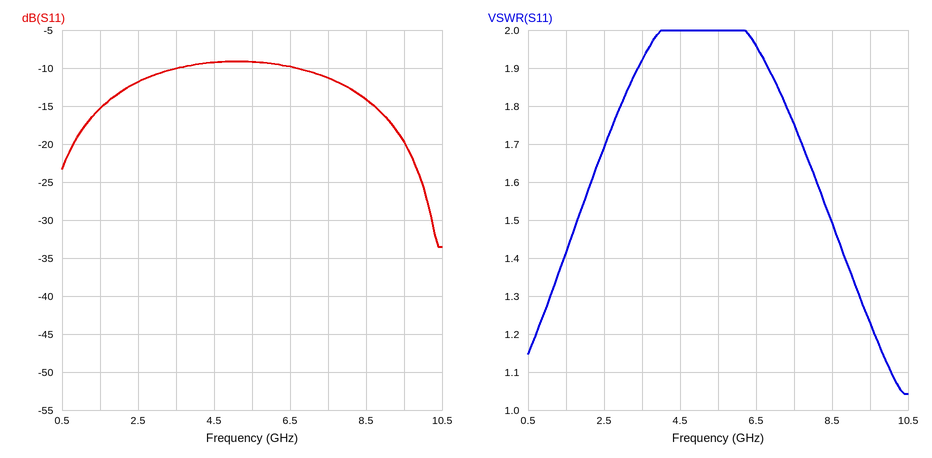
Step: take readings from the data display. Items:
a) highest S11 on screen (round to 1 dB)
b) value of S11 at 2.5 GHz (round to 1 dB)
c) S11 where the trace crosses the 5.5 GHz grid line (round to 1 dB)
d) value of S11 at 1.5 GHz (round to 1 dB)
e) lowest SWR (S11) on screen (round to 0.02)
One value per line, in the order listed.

-9 dB
-12 dB
-9 dB
-15 dB
1.04
